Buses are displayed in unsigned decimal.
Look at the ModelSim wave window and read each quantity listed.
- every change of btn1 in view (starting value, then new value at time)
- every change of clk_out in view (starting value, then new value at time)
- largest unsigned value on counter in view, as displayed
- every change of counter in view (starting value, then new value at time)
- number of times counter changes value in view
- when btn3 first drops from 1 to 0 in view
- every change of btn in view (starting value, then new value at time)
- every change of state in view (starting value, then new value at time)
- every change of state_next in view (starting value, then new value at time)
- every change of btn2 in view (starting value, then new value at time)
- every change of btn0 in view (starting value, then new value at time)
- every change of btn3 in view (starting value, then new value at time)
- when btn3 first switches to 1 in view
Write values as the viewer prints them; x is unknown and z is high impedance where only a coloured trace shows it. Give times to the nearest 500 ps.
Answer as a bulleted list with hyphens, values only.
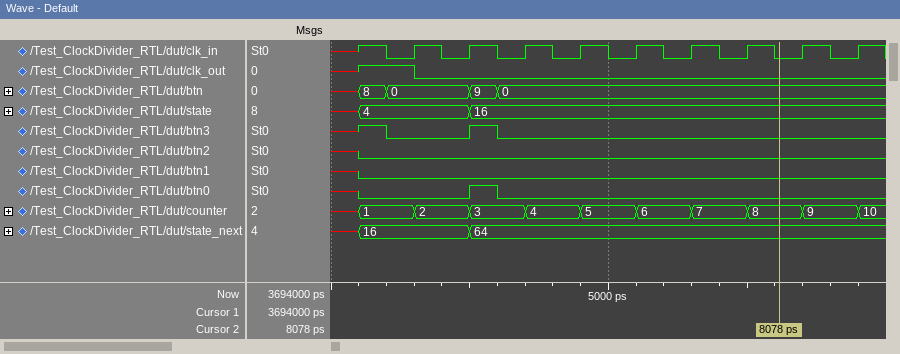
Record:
- x, 0 at 500 ps
- x, 1 at 500 ps, 0 at 1500 ps
- 10
- x, 1 at 500 ps, 2 at 1500 ps, 3 at 2500 ps, 4 at 3500 ps, 5 at 4500 ps, 6 at 5500 ps, 7 at 6500 ps, 8 at 7500 ps, 9 at 8500 ps, 10 at 9500 ps
- 10
- 1000 ps
- x, 8 at 500 ps, 0 at 1000 ps, 9 at 2500 ps, 0 at 3000 ps
- x, 4 at 500 ps, 16 at 2500 ps
- x, 16 at 500 ps, 64 at 2500 ps
- x, 0 at 500 ps
- x, 0 at 500 ps, 1 at 2500 ps, 0 at 3000 ps
- x, 1 at 500 ps, 0 at 1000 ps, 1 at 2500 ps, 0 at 3000 ps
- 500 ps
